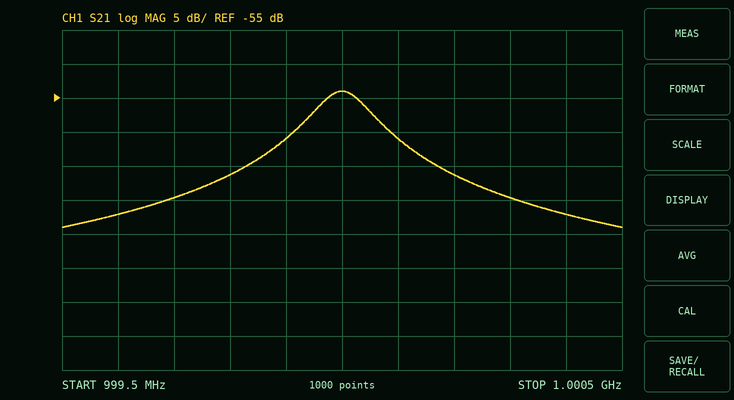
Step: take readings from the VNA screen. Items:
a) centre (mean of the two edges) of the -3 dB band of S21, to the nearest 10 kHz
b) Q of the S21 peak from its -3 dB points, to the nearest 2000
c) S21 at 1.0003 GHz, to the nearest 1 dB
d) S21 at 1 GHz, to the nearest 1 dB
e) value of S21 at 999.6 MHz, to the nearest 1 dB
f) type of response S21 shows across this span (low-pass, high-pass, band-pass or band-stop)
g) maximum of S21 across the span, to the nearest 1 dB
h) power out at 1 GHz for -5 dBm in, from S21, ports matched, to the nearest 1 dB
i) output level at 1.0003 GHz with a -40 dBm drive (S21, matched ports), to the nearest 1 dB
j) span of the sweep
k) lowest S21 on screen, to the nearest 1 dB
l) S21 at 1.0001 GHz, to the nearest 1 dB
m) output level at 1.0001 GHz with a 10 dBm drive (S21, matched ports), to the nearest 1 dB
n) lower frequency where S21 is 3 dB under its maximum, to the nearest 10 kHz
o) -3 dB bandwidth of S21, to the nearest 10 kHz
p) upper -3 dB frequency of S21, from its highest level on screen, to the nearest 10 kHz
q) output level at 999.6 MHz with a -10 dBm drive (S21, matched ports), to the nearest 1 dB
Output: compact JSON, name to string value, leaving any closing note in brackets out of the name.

{"centre (mean of the two edges) of the -3 dB band of S21, to the nearest 10 kHz": "1.00000 GHz", "Q of the S21 peak from its -3 dB points, to the nearest 2000": "10000", "S21 at 1.0003 GHz, to the nearest 1 dB": "-70 dB", "S21 at 1 GHz, to the nearest 1 dB": "-54 dB", "value of S21 at 999.6 MHz, to the nearest 1 dB": "-72 dB", "type of response S21 shows across this span": "band-pass", "maximum of S21 across the span, to the nearest 1 dB": "-54 dB", "power out at 1 GHz for -5 dBm in, from S21, ports matched, to the nearest 1 dB": "-59 dBm", "output level at 1.0003 GHz with a -40 dBm drive (S21, matched ports), to the nearest 1 dB": "-110 dBm", "span of the sweep": "1 MHz", "lowest S21 on screen, to the nearest 1 dB": "-74 dB", "S21 at 1.0001 GHz, to the nearest 1 dB": "-61 dB", "output level at 1.0001 GHz with a 10 dBm drive (S21, matched ports), to the nearest 1 dB": "-51 dBm", "lower frequency where S21 is 3 dB under its maximum, to the nearest 10 kHz": "999.95 MHz", "-3 dB bandwidth of S21, to the nearest 10 kHz": "100 kHz", "upper -3 dB frequency of S21, from its highest level on screen, to the nearest 10 kHz": "1.00005 GHz", "output level at 999.6 MHz with a -10 dBm drive (S21, matched ports), to the nearest 1 dB": "-82 dBm"}
